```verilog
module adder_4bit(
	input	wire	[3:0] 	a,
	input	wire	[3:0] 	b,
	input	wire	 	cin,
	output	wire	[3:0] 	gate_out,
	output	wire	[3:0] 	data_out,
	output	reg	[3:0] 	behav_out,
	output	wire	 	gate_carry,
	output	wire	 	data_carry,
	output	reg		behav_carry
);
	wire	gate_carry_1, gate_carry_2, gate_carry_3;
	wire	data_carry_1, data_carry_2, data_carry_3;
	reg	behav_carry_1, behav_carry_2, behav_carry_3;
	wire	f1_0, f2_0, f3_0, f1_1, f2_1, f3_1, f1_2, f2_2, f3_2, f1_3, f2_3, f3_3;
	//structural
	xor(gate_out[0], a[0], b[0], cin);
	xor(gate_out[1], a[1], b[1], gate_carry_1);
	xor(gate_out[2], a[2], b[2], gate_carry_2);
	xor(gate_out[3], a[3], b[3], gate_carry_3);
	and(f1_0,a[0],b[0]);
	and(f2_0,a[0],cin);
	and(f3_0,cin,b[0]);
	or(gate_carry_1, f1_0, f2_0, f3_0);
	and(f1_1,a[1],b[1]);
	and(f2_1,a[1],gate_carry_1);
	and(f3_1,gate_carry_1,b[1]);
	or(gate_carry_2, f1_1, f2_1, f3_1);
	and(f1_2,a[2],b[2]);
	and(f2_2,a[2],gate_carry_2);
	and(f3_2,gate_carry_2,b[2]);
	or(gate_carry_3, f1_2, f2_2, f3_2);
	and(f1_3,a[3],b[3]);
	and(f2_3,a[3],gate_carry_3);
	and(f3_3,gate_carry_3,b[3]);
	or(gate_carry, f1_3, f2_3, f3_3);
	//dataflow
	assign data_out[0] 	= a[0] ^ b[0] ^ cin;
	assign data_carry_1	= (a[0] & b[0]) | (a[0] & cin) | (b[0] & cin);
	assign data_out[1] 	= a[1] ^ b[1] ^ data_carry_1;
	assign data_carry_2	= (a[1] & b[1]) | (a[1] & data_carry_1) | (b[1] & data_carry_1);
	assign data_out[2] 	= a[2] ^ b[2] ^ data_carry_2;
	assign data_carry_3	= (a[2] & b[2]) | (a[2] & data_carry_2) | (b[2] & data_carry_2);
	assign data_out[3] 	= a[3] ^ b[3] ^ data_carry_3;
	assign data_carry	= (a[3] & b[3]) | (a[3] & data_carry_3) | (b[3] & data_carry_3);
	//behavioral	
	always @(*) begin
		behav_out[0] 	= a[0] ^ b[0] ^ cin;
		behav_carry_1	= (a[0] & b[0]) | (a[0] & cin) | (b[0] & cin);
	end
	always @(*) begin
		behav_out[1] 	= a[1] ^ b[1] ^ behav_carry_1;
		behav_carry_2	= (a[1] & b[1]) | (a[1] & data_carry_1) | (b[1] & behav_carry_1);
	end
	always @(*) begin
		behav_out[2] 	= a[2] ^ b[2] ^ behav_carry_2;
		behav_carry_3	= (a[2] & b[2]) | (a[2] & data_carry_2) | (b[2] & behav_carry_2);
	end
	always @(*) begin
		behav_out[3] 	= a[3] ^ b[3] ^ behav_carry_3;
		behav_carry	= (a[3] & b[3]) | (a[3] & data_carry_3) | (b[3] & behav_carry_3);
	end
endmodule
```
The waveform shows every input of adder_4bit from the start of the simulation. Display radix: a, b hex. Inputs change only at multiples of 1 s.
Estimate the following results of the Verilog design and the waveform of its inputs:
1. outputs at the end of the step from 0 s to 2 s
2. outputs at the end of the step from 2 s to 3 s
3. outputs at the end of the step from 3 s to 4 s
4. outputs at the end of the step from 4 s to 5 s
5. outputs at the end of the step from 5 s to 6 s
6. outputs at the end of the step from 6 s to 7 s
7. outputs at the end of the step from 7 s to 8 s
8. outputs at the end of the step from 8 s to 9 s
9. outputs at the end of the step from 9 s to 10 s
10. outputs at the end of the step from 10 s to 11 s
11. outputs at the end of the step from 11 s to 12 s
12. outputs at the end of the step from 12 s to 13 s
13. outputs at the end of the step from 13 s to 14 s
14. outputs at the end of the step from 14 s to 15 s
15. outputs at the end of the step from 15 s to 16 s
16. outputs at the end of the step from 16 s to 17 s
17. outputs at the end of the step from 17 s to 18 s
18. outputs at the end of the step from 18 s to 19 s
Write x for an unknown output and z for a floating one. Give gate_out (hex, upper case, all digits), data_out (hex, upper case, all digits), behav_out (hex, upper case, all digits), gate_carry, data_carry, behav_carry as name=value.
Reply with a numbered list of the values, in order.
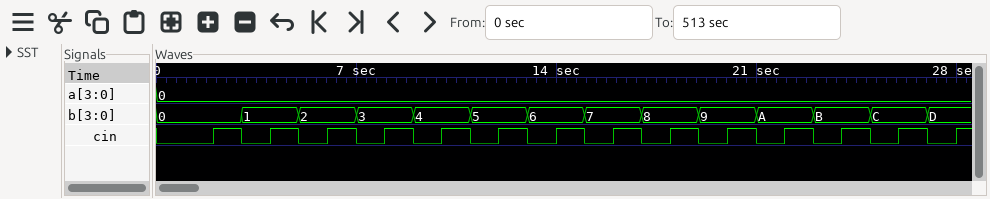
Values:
1. gate_out=0, data_out=0, behav_out=0, gate_carry=0, data_carry=0, behav_carry=0
2. gate_out=1, data_out=1, behav_out=1, gate_carry=0, data_carry=0, behav_carry=0
3. gate_out=1, data_out=1, behav_out=1, gate_carry=0, data_carry=0, behav_carry=0
4. gate_out=2, data_out=2, behav_out=2, gate_carry=0, data_carry=0, behav_carry=0
5. gate_out=2, data_out=2, behav_out=2, gate_carry=0, data_carry=0, behav_carry=0
6. gate_out=3, data_out=3, behav_out=3, gate_carry=0, data_carry=0, behav_carry=0
7. gate_out=3, data_out=3, behav_out=3, gate_carry=0, data_carry=0, behav_carry=0
8. gate_out=4, data_out=4, behav_out=4, gate_carry=0, data_carry=0, behav_carry=0
9. gate_out=4, data_out=4, behav_out=4, gate_carry=0, data_carry=0, behav_carry=0
10. gate_out=5, data_out=5, behav_out=5, gate_carry=0, data_carry=0, behav_carry=0
11. gate_out=5, data_out=5, behav_out=5, gate_carry=0, data_carry=0, behav_carry=0
12. gate_out=6, data_out=6, behav_out=6, gate_carry=0, data_carry=0, behav_carry=0
13. gate_out=6, data_out=6, behav_out=6, gate_carry=0, data_carry=0, behav_carry=0
14. gate_out=7, data_out=7, behav_out=7, gate_carry=0, data_carry=0, behav_carry=0
15. gate_out=7, data_out=7, behav_out=7, gate_carry=0, data_carry=0, behav_carry=0
16. gate_out=8, data_out=8, behav_out=8, gate_carry=0, data_carry=0, behav_carry=0
17. gate_out=8, data_out=8, behav_out=8, gate_carry=0, data_carry=0, behav_carry=0
18. gate_out=9, data_out=9, behav_out=9, gate_carry=0, data_carry=0, behav_carry=0
